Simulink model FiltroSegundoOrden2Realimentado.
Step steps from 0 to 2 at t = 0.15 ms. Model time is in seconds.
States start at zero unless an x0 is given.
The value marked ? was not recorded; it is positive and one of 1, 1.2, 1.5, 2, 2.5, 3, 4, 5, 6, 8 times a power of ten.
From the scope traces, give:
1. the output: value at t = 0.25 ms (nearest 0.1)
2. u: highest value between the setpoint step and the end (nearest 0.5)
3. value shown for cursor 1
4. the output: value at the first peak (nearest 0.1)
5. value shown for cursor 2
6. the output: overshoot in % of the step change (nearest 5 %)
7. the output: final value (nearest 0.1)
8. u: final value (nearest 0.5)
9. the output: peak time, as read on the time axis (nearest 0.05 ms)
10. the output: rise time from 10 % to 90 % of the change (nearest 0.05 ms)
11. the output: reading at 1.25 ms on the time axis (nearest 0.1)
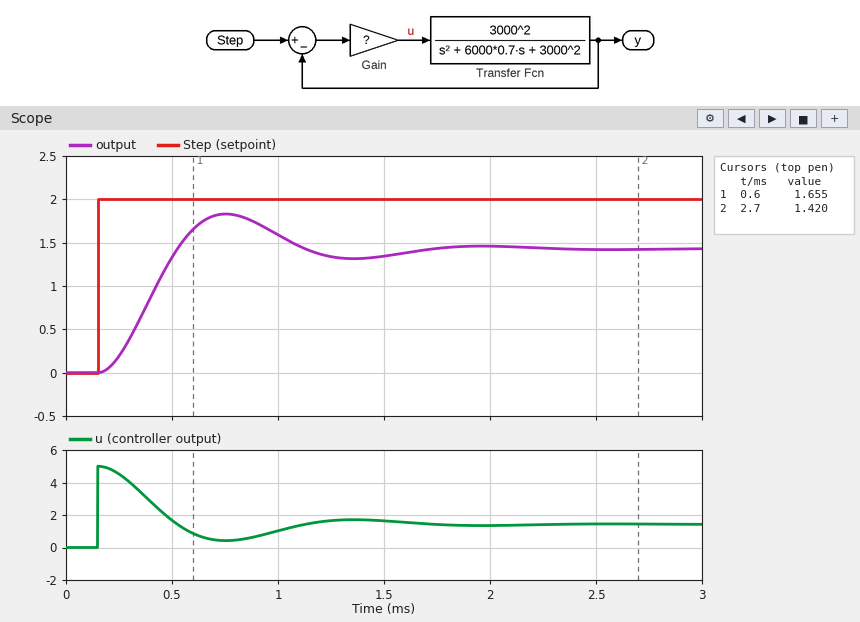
0.2
5.0
1.655
1.8
1.420
30 %
1.4
1.5
0.75 ms
0.25 ms
1.3
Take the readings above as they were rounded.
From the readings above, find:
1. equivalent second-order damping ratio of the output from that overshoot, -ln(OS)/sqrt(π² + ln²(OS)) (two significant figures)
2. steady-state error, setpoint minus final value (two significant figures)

0.36
0.60
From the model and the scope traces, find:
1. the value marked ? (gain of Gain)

2.5
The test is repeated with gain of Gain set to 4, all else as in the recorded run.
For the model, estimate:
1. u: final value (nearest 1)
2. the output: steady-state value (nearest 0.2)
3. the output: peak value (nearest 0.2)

2
1.6
2.2
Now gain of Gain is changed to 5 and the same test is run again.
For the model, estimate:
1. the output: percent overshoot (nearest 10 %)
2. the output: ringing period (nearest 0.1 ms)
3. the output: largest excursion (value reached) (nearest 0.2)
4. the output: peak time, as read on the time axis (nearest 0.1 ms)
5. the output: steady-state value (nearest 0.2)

40 %
0.9 ms
2.4
0.6 ms
1.6
